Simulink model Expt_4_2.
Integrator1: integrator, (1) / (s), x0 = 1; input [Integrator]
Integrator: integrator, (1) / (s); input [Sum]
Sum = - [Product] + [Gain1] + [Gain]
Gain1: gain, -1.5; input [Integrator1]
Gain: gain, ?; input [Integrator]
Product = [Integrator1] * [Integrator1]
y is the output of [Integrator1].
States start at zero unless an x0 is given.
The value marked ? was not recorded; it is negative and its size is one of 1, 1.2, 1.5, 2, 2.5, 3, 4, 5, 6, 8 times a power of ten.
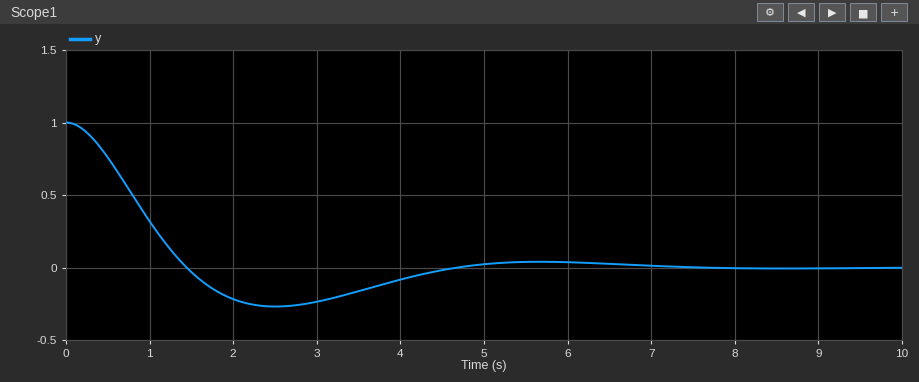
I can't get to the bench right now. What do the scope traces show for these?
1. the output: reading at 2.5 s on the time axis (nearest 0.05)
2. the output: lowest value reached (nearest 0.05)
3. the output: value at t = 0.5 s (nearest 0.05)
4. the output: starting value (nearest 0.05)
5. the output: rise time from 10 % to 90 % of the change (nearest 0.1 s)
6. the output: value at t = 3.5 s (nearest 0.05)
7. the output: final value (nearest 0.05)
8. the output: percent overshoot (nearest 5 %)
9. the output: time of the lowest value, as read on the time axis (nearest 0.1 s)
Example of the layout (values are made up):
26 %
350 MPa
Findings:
-0.25
-0.25
0.75
1.00
1.0 s
-0.15
0.00
25 %
2.5 s
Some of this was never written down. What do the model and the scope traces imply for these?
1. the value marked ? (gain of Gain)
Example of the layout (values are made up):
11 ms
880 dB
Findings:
-1.2
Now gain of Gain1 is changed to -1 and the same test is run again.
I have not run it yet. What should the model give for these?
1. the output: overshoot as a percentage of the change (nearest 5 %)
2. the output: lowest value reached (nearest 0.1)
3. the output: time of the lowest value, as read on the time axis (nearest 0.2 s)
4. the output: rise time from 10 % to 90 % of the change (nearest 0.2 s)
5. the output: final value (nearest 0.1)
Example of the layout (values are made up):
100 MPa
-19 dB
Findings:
20 %
-0.2
3.0 s
1.2 s
0.0
